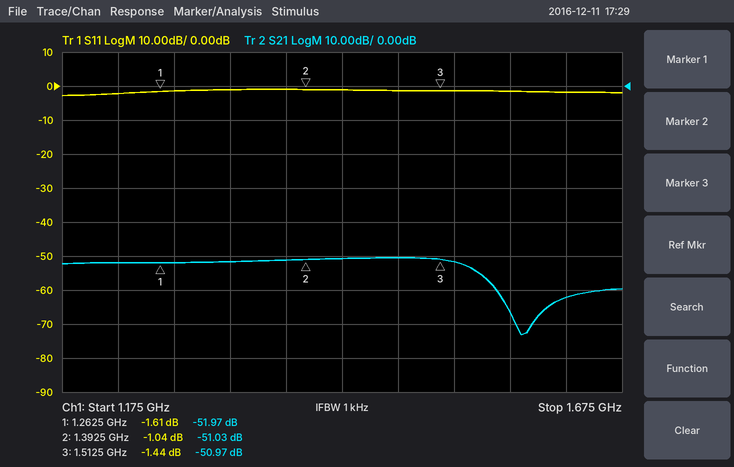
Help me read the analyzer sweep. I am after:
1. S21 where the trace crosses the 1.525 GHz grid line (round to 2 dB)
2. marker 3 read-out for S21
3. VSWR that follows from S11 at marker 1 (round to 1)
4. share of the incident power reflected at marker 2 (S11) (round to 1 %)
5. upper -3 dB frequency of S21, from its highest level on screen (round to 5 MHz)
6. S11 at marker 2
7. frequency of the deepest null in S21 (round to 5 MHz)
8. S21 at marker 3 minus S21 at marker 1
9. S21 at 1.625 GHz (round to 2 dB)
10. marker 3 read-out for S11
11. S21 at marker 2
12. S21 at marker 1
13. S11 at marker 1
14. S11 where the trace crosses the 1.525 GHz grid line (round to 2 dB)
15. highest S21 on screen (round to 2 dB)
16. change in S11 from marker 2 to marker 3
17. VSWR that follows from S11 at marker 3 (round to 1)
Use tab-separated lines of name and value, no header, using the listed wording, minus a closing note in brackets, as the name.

S21 where the trace crosses the 1.525 GHz grid line	-52 dB
marker 3 read-out for S21	-50.97 dB
VSWR that follows from S11 at marker 1	11
share of the incident power reflected at marker 2 (S11)	79 %
upper -3 dB frequency of S21, from its highest level on screen	1.540 GHz
S11 at marker 2	-1.04 dB
frequency of the deepest null in S21	1.585 GHz
S21 at marker 3 minus S21 at marker 1	1.00 dB
S21 at 1.625 GHz	-62 dB
marker 3 read-out for S11	-1.44 dB
S21 at marker 2	-51.03 dB
S21 at marker 1	-51.97 dB
S11 at marker 1	-1.61 dB
S11 where the trace crosses the 1.525 GHz grid line	-2 dB
highest S21 on screen	-50 dB
change in S11 from marker 2 to marker 3	-0.40 dB
VSWR that follows from S11 at marker 3	12
